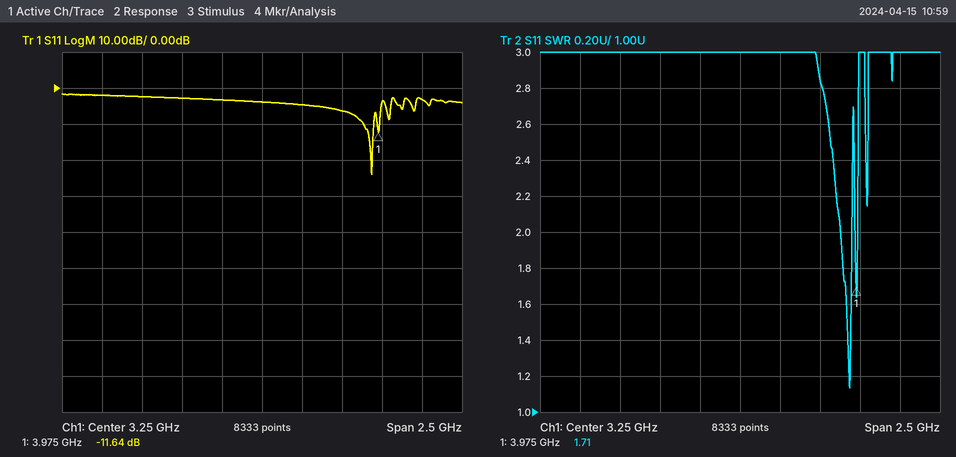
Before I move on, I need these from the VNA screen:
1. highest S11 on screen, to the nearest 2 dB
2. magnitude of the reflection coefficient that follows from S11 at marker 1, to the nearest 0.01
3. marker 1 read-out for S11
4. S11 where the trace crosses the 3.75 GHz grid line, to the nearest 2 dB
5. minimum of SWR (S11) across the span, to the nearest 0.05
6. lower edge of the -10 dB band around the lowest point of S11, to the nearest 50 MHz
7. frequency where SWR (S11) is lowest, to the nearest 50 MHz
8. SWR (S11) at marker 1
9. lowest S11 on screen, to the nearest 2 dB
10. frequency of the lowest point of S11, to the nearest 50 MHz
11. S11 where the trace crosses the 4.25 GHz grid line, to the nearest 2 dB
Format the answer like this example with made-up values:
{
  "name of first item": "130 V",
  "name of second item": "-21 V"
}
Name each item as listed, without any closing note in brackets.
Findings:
{
  "highest S11 on screen, to the nearest 2 dB": "-2 dB",
  "magnitude of the reflection coefficient that follows from S11 at marker 1, to the nearest 0.01": "0.26",
  "marker 1 read-out for S11": "-11.64 dB",
  "S11 where the trace crosses the 3.75 GHz grid line, to the nearest 2 dB": "-6 dB",
  "minimum of SWR (S11) across the span, to the nearest 0.05": "1.15",
  "lower edge of the -10 dB band around the lowest point of S11, to the nearest 50 MHz": "3.90 GHz",
  "frequency where SWR (S11) is lowest, to the nearest 50 MHz": "3.95 GHz",
  "SWR (S11) at marker 1": "1.71",
  "lowest S11 on screen, to the nearest 2 dB": "-24 dB",
  "frequency of the lowest point of S11, to the nearest 50 MHz": "3.95 GHz",
  "S11 where the trace crosses the 4.25 GHz grid line, to the nearest 2 dB": "-4 dB"
}
